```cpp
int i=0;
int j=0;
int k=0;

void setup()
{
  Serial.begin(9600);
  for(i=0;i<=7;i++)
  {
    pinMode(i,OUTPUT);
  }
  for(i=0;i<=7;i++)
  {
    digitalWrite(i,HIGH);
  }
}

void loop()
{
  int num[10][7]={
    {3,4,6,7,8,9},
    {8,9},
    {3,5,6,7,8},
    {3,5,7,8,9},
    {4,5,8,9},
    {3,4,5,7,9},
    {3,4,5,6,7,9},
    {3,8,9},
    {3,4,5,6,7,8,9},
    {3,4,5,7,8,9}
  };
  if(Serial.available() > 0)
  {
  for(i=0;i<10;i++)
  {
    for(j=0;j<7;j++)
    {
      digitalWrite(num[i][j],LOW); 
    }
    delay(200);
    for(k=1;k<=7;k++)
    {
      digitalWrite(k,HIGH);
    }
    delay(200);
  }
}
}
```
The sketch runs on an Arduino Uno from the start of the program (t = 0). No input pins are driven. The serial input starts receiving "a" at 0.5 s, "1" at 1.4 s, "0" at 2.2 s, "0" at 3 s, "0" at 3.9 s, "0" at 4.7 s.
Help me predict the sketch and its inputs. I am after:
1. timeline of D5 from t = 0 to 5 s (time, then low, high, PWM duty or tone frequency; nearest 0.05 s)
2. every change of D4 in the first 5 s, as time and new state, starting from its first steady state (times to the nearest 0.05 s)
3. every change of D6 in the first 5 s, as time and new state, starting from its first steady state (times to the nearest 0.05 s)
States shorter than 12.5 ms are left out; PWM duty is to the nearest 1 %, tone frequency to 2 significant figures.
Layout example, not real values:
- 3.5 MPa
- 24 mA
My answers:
- 0 s high; 1.3 s low; 1.5 s high; 1.7 s low; 1.9 s high; 2.1 s low; 2.3 s high; 2.5 s low; 2.7 s high; 2.9 s low; 3.1 s high; 3.7 s low; 3.9 s high; 4.1 s low; 4.3 s high
- 0 s high; 0.5 s low; 0.7 s high; 2.1 s low; 2.3 s high; 2.5 s low; 2.7 s high; 2.9 s low; 3.1 s high; 3.7 s low; 3.9 s high; 4.1 s low; 4.3 s high; 4.5 s low; 4.7 s high
- 0 s high; 0.5 s low; 0.7 s high; 1.3 s low; 1.5 s high; 2.9 s low; 3.1 s high; 3.7 s low; 3.9 s high; 4.5 s low; 4.7 s high
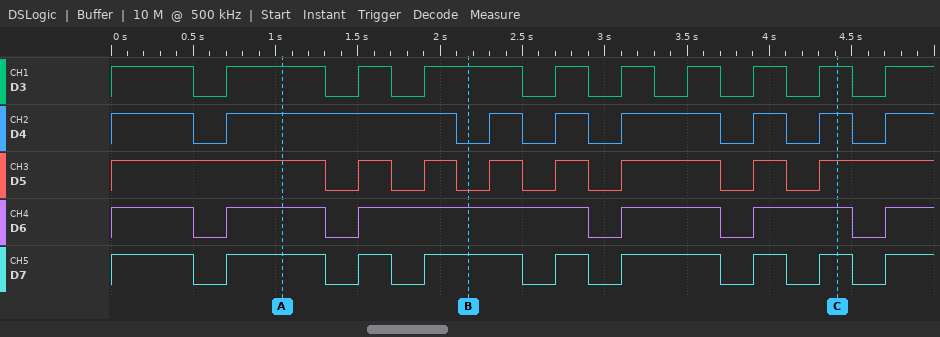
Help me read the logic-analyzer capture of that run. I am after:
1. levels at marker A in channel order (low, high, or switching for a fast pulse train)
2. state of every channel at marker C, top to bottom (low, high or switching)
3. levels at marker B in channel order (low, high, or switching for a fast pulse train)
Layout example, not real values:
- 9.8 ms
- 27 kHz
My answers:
- D3 high, D4 high, D5 high, D6 high, D7 high
- D3 high, D4 high, D5 high, D6 high, D7 high
- D3 high, D4 low, D5 low, D6 high, D7 high
